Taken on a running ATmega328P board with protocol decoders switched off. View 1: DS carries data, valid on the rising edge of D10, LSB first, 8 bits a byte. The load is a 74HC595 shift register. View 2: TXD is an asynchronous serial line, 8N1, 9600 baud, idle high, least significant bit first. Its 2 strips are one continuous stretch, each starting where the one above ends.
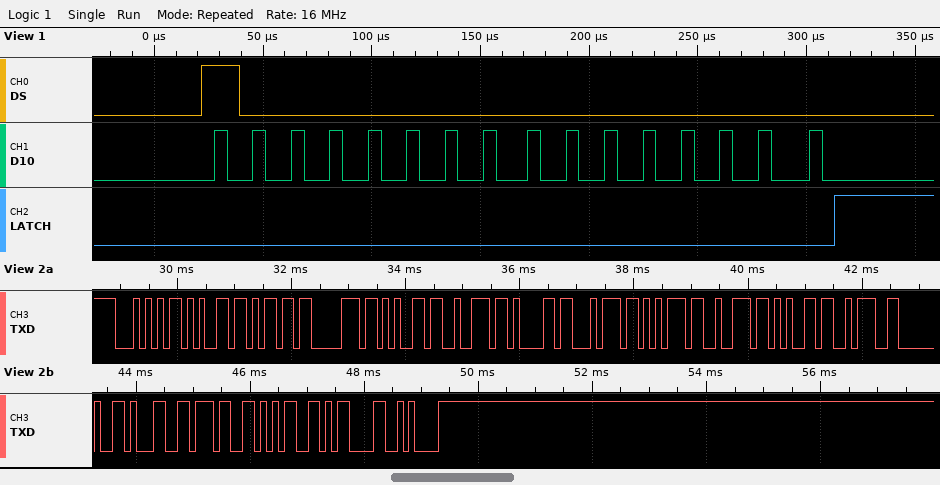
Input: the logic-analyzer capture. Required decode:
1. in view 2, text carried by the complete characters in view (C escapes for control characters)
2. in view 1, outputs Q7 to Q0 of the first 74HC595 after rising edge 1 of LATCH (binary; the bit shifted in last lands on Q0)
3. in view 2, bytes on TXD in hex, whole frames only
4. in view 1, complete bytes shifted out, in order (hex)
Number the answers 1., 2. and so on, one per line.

1. "Temperature: 175\r\n"
2. 00000000
3. 54 65 6D 70 65 72 61 74 75 72 65 3A 20 31 37 35 0D 0A
4. 01 00
